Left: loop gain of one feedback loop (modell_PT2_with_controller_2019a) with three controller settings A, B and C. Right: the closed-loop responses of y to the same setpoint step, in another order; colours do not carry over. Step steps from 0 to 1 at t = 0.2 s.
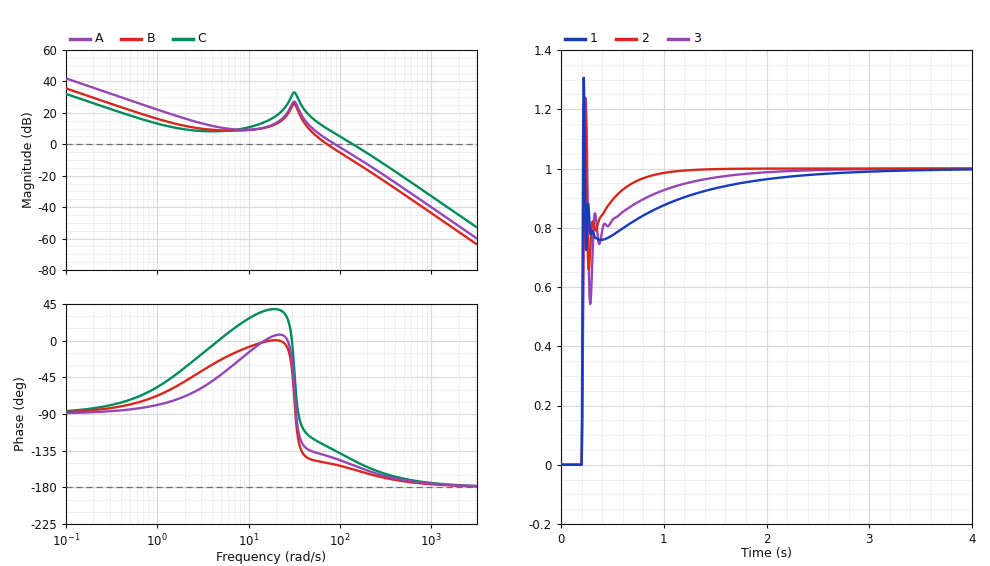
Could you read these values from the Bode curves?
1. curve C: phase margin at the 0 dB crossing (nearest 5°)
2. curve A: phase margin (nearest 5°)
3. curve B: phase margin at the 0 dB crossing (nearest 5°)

35°
35°
30°
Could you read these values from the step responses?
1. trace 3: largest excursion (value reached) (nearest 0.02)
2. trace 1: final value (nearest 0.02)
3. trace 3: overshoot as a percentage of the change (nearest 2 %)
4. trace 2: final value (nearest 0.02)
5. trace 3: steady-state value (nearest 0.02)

1.24
1.00
24 %
1.00
1.00
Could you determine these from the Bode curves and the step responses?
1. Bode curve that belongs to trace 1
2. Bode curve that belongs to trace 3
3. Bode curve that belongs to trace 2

C
B
A
